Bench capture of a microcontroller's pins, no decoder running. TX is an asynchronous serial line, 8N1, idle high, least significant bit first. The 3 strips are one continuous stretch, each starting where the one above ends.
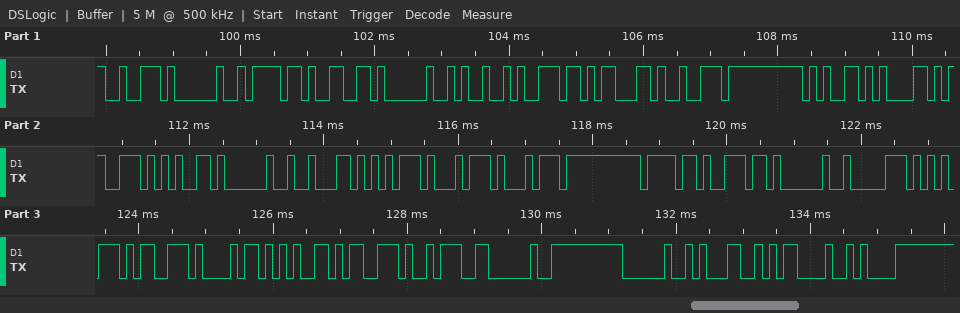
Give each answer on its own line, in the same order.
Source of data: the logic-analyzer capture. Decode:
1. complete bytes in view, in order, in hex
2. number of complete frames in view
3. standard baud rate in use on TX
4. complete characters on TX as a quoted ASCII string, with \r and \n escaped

72 20 6F 66 20 49 6E 63 72 65 61 73 65 20 62 75 74 74 6F 6E 20 70 75 73 68 65 73 3A 20 20 31 0D 0A
33
9600 baud
"r of Increase button pushes:  1\r\n"
